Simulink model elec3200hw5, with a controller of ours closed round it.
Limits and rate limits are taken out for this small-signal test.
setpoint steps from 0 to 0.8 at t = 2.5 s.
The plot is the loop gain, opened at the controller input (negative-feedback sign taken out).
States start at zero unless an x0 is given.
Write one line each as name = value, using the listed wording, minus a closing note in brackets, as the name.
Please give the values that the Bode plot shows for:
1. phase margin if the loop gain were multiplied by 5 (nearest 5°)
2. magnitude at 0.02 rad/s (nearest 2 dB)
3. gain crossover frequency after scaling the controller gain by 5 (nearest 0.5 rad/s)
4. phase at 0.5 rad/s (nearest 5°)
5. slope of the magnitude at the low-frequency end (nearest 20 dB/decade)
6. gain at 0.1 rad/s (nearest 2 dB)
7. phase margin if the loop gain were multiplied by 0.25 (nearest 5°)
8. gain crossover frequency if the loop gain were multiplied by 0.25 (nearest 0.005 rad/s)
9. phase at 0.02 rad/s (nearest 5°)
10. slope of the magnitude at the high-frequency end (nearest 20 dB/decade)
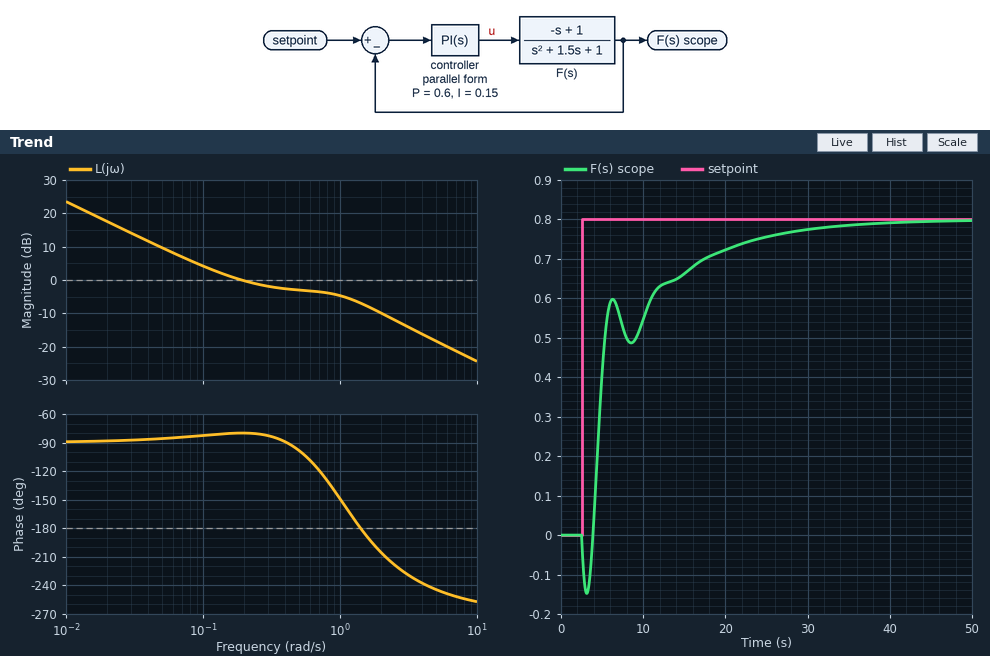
phase margin if the loop gain were multiplied by 5 = -50°
magnitude at 0.02 rad/s = 18 dB
gain crossover frequency after scaling the controller gain by 5 = 3.0 rad/s
phase at 0.5 rad/s = -100°
slope of the magnitude at the low-frequency end = -20 dB/decade
gain at 0.1 rad/s = 4 dB
phase margin if the loop gain were multiplied by 0.25 = 95°
gain crossover frequency if the loop gain were multiplied by 0.25 = 0.040 rad/s
phase at 0.02 rad/s = -90°
slope of the magnitude at the high-frequency end = -20 dB/decade
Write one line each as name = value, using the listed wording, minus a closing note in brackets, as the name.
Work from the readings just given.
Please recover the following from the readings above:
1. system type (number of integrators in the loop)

system type = 1
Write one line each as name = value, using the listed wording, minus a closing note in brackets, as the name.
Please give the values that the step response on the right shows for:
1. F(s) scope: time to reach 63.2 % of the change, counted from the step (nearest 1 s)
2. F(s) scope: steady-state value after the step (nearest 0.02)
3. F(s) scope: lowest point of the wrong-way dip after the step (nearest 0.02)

F(s) scope: time to reach 63.2 % of the change, counted from the step = 3 s
F(s) scope: steady-state value after the step = 0.80
F(s) scope: lowest point of the wrong-way dip after the step = -0.14
